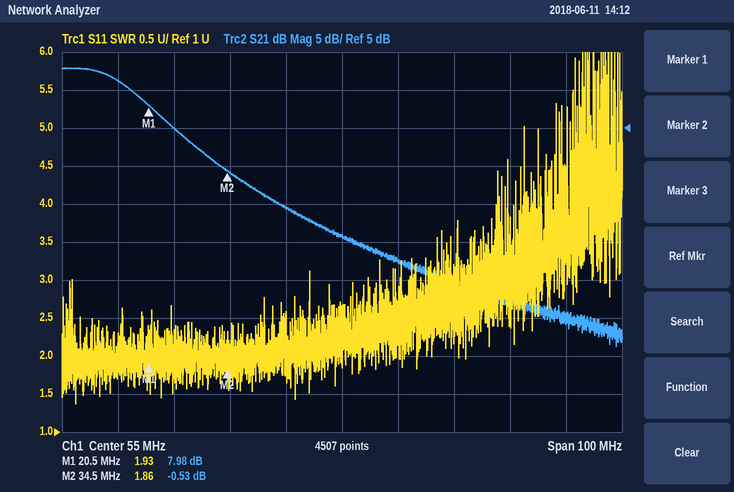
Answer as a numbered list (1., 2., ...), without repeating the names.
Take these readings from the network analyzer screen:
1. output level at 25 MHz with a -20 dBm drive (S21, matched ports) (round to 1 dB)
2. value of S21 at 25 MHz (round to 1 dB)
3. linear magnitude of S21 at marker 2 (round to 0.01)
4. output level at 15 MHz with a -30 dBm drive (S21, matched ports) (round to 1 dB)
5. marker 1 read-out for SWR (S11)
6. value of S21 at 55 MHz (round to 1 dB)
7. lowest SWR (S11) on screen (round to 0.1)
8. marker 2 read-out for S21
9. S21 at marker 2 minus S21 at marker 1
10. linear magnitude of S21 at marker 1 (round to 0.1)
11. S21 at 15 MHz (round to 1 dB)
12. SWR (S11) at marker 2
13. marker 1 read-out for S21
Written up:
1. -15 dBm
2. 5 dB
3. 0.94
4. -19 dBm
5. 1.93
6. -9 dB
7. 1.4
8. -0.53 dB
9. -8.51 dB
10. 2.5
11. 11 dB
12. 1.86
13. 7.98 dB
